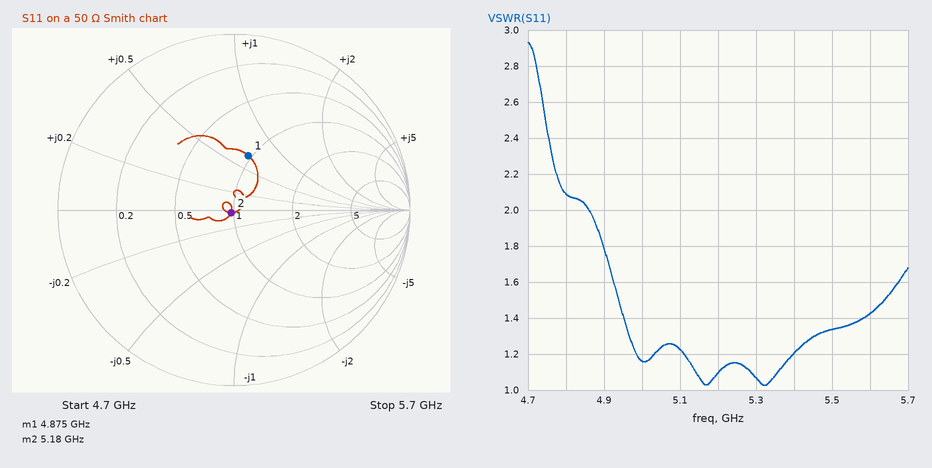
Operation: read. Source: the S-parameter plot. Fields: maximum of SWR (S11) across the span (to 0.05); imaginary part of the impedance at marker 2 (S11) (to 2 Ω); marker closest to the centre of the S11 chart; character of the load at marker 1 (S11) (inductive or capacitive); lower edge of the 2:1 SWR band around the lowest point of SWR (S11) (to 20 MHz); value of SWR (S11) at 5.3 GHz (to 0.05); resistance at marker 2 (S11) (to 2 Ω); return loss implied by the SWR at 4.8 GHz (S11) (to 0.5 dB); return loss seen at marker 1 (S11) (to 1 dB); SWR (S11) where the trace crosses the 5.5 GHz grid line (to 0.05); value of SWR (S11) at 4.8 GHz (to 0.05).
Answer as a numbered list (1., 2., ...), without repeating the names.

1. 2.95
2. -2 Ω
3. marker 2
4. inductive
5. 4.86 GHz
6. 1.05
7. 48 Ω
8. 9.0 dB
9. 10 dB
10. 1.35
11. 2.10
